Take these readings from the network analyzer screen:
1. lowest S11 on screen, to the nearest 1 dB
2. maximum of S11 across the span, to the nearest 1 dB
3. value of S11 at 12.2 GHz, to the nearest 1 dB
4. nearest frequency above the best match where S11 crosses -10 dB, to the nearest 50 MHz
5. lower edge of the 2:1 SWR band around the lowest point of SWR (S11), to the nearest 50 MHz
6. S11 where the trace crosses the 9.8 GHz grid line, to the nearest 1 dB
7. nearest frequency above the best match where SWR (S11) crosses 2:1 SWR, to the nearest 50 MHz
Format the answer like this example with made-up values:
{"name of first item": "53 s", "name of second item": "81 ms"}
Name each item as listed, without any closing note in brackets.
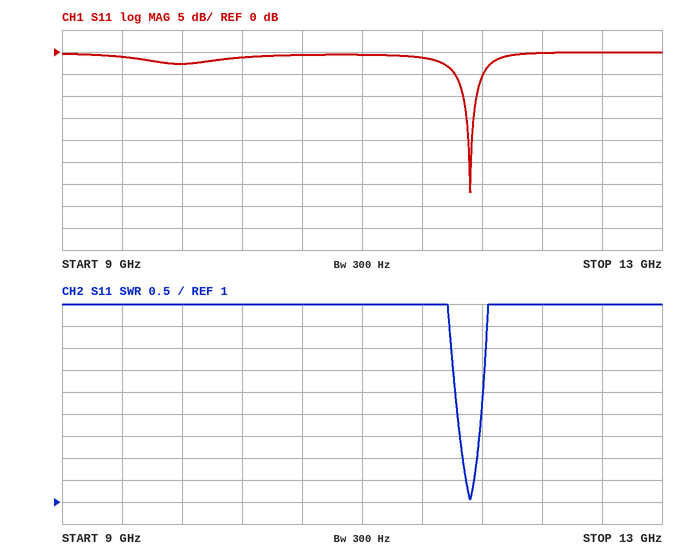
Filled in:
{"lowest S11 on screen, to the nearest 1 dB": "-32 dB", "maximum of S11 across the span, to the nearest 1 dB": "0 dB", "value of S11 at 12.2 GHz, to the nearest 1 dB": "0 dB", "nearest frequency above the best match where S11 crosses -10 dB, to the nearest 50 MHz": "11.75 GHz", "lower edge of the 2:1 SWR band around the lowest point of SWR (S11), to the nearest 50 MHz": "11.65 GHz", "S11 where the trace crosses the 9.8 GHz grid line, to the nearest 1 dB": "-3 dB", "nearest frequency above the best match where SWR (S11) crosses 2:1 SWR, to the nearest 50 MHz": "11.75 GHz"}
